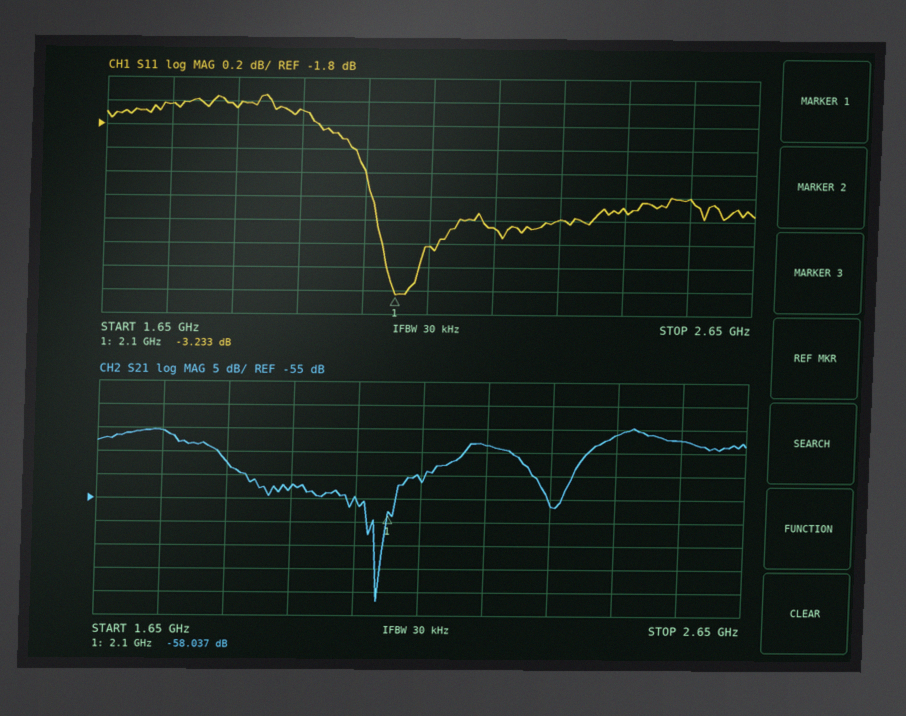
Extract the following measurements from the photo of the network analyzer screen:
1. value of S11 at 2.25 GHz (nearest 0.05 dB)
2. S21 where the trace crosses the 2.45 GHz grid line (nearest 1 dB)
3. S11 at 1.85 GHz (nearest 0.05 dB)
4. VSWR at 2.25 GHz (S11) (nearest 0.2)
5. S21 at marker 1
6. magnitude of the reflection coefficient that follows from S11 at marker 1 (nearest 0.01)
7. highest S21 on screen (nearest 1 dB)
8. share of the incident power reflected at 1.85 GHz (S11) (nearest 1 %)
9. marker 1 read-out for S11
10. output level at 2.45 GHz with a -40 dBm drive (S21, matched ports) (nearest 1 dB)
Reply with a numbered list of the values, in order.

1. -2.65 dB
2. -41 dB
3. -1.65 dB
4. 6.6
5. -58.037 dB
6. 0.69
7. -40 dB
8. 68 %
9. -3.233 dB
10. -81 dBm
